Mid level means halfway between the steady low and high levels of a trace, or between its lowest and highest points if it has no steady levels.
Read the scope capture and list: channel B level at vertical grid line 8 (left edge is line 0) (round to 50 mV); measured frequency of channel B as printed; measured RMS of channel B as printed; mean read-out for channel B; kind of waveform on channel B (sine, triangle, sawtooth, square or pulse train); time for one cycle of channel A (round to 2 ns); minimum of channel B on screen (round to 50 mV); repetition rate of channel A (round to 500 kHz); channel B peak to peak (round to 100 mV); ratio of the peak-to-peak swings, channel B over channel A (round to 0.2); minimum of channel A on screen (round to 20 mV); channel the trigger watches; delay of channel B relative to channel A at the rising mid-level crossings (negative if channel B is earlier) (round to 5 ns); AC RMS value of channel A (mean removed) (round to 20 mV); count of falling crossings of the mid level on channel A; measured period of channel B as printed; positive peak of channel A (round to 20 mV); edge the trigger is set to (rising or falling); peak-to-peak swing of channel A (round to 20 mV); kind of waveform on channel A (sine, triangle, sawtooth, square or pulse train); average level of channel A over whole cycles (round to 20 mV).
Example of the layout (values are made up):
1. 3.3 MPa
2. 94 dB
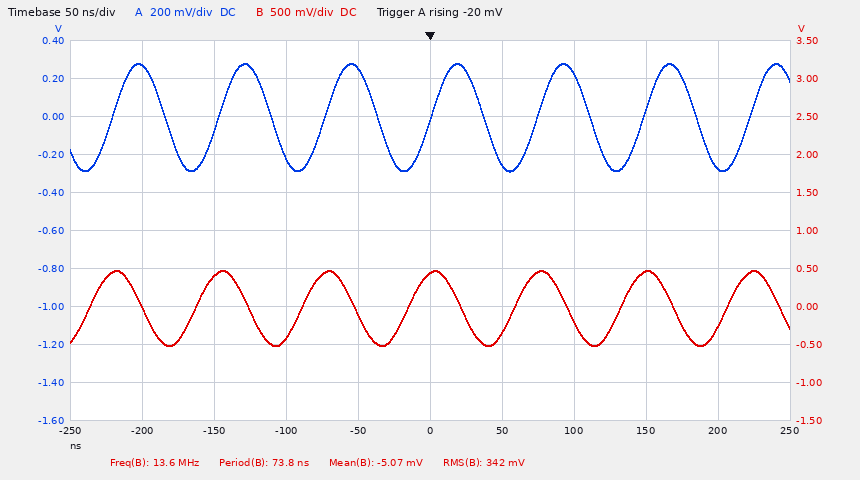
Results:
1. 450 mV
2. 13.6 MHz
3. 342 mV
4. -5.07 mV
5. sine
6. 74 ns
7. -500 mV
8. 13.5 MHz
9. 1.00 V
10. 1.8
11. -280 mV
12. channel A
13. -15 ns
14. 200 mV
15. 6
16. 73.8 ns
17. 280 mV
18. rising
19. 560 mV
20. sine
21. 0 mV
